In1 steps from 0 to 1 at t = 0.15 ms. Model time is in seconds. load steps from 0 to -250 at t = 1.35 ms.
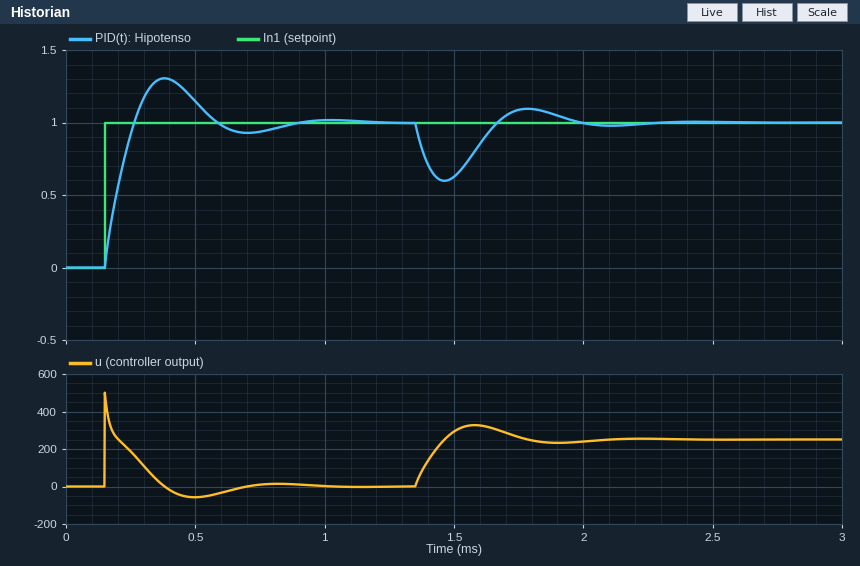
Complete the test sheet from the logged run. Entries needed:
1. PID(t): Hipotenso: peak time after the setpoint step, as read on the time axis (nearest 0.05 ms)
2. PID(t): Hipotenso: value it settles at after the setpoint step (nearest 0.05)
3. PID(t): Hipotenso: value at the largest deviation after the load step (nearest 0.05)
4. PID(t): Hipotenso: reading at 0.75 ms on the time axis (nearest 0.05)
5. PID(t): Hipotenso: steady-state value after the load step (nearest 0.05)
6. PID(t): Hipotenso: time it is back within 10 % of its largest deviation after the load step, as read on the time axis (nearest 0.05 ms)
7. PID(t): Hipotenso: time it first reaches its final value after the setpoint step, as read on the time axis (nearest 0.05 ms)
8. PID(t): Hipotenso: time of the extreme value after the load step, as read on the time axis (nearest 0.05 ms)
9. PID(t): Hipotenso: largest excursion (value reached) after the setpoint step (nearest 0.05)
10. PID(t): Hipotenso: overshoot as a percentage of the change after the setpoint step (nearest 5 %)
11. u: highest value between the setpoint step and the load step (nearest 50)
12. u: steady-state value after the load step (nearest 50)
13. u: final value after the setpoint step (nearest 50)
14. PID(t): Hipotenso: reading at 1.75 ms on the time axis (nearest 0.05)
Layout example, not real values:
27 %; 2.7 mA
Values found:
0.40 ms; 1.00; 0.60; 0.95; 1.00; 1.90 ms; 0.25 ms; 1.45 ms; 1.30; 30 %; 500; 250; 0; 1.10
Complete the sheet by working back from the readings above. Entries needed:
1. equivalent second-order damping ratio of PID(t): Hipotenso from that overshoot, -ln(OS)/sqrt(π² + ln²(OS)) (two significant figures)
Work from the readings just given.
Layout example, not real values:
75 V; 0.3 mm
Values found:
0.36
